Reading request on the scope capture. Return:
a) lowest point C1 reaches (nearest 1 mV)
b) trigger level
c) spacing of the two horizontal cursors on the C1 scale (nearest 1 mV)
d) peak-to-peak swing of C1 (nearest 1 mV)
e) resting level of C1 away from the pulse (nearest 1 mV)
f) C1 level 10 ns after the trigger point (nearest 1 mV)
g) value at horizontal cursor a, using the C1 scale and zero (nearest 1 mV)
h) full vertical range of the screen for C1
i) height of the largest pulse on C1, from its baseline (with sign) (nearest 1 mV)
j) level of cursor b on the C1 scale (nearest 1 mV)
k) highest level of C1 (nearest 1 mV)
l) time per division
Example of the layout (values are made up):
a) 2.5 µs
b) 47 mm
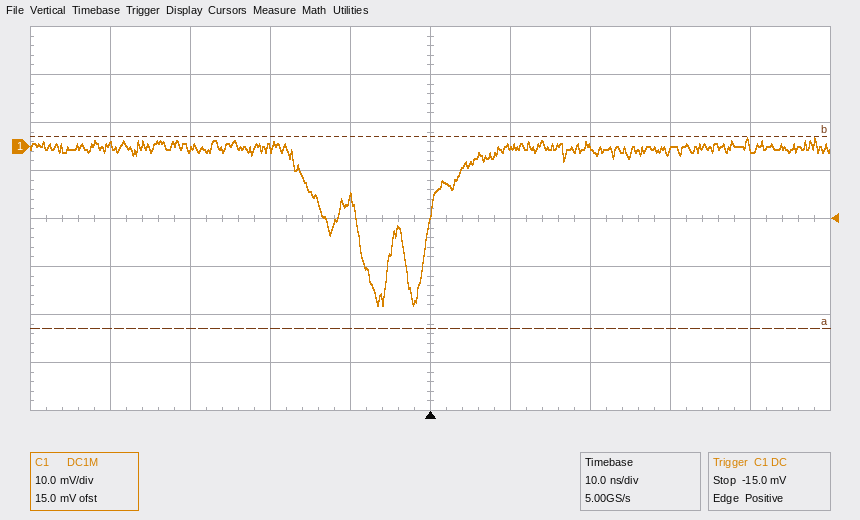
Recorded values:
a) -33 mV
b) -15.0 mV
c) 40 mV
d) 35 mV
e) 0 mV
f) 0 mV
g) -38 mV
h) 80 mV
i) -33 mV
j) 2 mV
k) 2 mV
l) 10 ns
